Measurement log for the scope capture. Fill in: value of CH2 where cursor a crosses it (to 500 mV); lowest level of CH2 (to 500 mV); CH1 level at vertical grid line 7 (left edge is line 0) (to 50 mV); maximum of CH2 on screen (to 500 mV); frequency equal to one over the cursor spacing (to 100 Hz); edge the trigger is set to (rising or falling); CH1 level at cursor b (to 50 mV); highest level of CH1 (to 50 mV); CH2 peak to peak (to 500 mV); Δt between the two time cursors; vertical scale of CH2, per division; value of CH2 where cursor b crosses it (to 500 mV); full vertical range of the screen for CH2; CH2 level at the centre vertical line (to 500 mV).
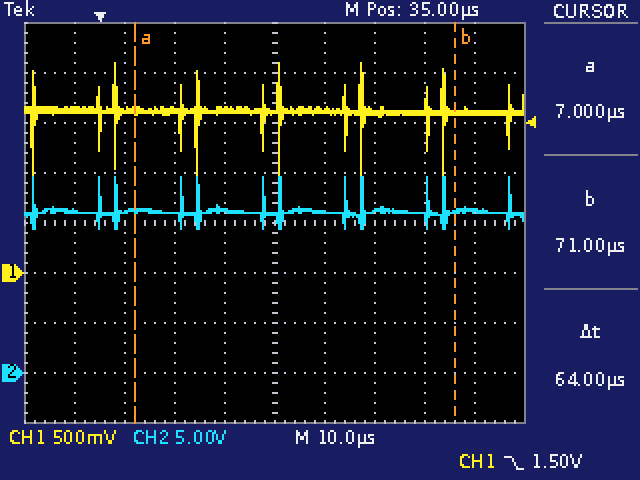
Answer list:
16.5 V
14.5 V
1.60 V
19.5 V
15.6 kHz
falling
1.60 V
2.10 V
5.0 V
64 µs
5 V
16.0 V
40 V
15.5 V
